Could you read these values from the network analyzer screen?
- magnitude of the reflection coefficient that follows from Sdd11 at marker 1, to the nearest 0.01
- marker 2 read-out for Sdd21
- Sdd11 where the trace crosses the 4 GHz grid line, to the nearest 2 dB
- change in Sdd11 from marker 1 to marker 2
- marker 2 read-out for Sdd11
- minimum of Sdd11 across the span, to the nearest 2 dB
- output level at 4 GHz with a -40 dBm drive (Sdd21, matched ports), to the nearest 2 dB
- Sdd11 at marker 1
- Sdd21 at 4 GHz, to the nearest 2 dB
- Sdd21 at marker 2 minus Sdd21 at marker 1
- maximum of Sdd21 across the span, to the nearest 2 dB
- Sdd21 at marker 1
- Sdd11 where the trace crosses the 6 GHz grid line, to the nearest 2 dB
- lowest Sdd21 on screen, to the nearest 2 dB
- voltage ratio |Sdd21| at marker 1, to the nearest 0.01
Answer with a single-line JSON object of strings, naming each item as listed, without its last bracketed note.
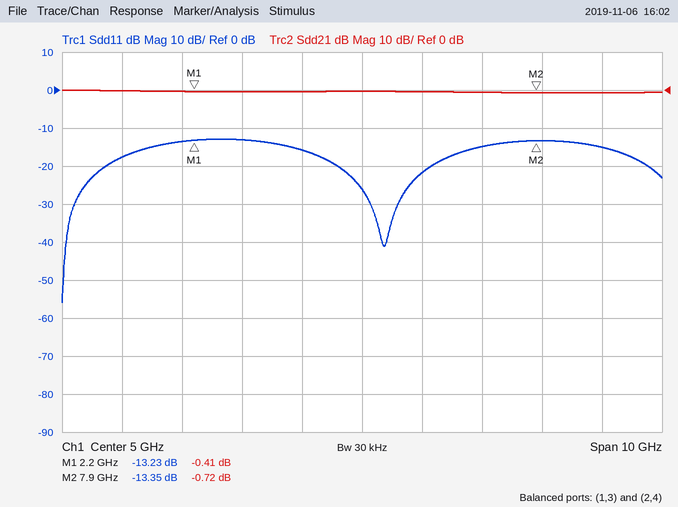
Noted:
{"magnitude of the reflection coefficient that follows from Sdd11 at marker 1, to the nearest 0.01": "0.22", "marker 2 read-out for Sdd21": "-0.72 dB", "Sdd11 where the trace crosses the 4 GHz grid line, to the nearest 2 dB": "-16 dB", "change in Sdd11 from marker 1 to marker 2": "-0.12 dB", "marker 2 read-out for Sdd11": "-13.35 dB", "minimum of Sdd11 across the span, to the nearest 2 dB": "-56 dB", "output level at 4 GHz with a -40 dBm drive (Sdd21, matched ports), to the nearest 2 dB": "-40 dBm", "Sdd11 at marker 1": "-13.23 dB", "Sdd21 at 4 GHz, to the nearest 2 dB": "0 dB", "Sdd21 at marker 2 minus Sdd21 at marker 1": "-0.31 dB", "maximum of Sdd21 across the span, to the nearest 2 dB": "0 dB", "Sdd21 at marker 1": "-0.41 dB", "Sdd11 where the trace crosses the 6 GHz grid line, to the nearest 2 dB": "-22 dB", "lowest Sdd21 on screen, to the nearest 2 dB": "0 dB", "voltage ratio |Sdd21| at marker 1, to the nearest 0.01": "0.95"}
